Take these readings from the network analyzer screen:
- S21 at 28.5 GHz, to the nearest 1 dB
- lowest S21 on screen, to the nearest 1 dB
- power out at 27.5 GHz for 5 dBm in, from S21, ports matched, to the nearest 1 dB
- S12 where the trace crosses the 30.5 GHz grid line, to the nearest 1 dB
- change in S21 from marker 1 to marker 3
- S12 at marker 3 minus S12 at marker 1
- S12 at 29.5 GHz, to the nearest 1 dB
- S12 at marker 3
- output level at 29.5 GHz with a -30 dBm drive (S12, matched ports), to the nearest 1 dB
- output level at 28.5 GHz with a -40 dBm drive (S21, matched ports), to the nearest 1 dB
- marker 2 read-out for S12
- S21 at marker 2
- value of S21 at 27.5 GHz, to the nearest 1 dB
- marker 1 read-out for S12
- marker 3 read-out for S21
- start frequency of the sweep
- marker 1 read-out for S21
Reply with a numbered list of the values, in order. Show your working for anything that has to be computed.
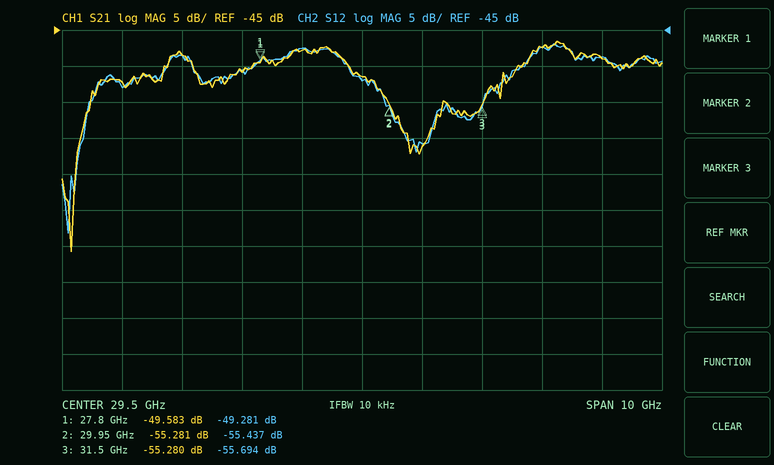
1. -48 dB
2. -76 dB
3. 5 dBm + (-51 dB) = -46 dBm
4. -61 dB
5. -55.28 − (-49.583) = -5.697 dB
6. -55.694 − (-49.281) = -6.413 dB
7. -52 dB
8. -55.694 dB
9. -30 dBm + (-52 dB) = -82 dBm
10. -40 dBm + (-48 dB) = -88 dBm
11. -55.437 dB
12. -55.281 dB
13. -51 dB
14. -49.281 dB
15. -55.280 dB
16. 24.5 GHz
17. -49.583 dB
